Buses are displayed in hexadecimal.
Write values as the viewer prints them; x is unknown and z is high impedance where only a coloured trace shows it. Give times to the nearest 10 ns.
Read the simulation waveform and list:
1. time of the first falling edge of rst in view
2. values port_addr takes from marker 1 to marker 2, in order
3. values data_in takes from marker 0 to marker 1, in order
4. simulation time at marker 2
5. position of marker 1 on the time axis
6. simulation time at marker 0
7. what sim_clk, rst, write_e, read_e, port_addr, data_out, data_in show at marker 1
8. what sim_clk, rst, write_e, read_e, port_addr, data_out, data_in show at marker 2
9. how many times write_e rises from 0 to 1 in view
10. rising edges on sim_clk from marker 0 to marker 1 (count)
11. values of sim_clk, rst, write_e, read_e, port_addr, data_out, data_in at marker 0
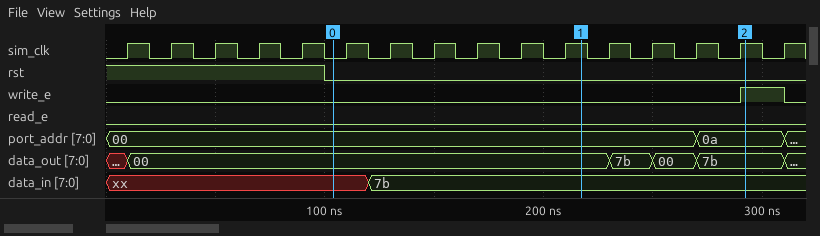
100 ns
00, 0a
xx, 7b
290 ns
220 ns
100 ns
sim_clk=1, rst=0, write_e=0, read_e=0, port_addr=00, data_out=00, data_in=7b
sim_clk=1, rst=0, write_e=1, read_e=0, port_addr=0a, data_out=7b, data_in=7b
1
6
sim_clk=0, rst=0, write_e=0, read_e=0, port_addr=00, data_out=00, data_in=xx
